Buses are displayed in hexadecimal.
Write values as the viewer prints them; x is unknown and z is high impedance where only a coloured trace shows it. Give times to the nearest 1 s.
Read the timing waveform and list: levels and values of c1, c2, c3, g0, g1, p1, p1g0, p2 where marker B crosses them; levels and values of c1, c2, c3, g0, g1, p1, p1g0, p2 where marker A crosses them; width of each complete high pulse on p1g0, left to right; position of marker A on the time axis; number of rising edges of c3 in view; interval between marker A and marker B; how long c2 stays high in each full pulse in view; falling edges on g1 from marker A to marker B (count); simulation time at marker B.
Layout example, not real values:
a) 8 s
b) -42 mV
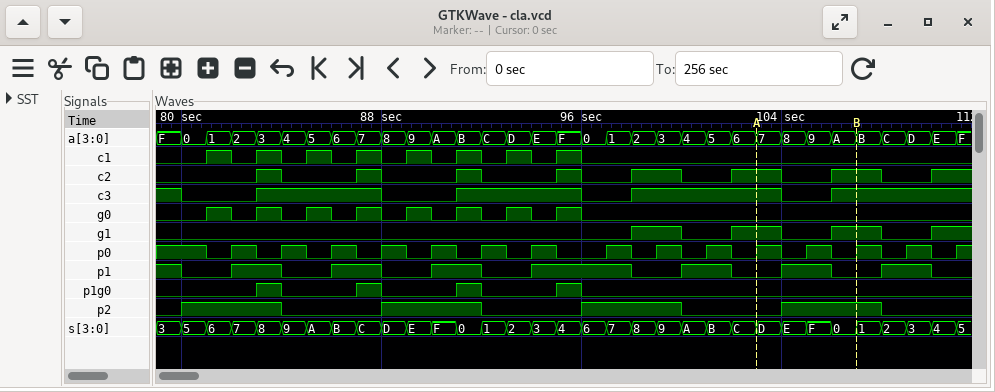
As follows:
a) c1=0, c2=1, c3=1, g0=0, g1=1, p1=0, p1g0=0, p2=1
b) c1=0, c2=1, c3=1, g0=0, g1=1, p1=0, p1g0=0, p2=0
c) 1 s, 1 s, 1 s, 1 s
d) 103 s
e) 4
f) 4 s
g) 1 s, 1 s, 1 s, 1 s, 2 s, 2 s, 2 s
h) 1
i) 107 s
